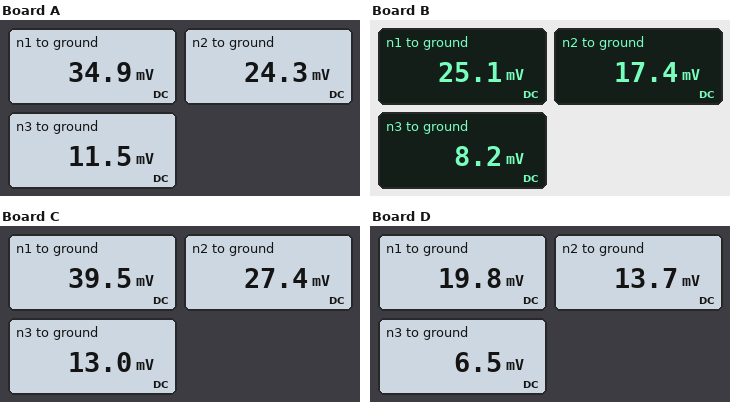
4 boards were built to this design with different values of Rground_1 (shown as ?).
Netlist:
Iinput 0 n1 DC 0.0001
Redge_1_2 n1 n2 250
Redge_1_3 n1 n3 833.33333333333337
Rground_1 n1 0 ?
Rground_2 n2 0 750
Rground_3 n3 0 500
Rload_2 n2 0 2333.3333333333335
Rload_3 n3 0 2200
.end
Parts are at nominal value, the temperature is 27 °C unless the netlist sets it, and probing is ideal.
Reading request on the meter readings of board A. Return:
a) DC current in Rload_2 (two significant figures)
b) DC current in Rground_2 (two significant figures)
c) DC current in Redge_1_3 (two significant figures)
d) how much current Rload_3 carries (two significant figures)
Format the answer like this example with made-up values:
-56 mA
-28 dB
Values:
10 µA
32 µA
28 µA
5.2 µA
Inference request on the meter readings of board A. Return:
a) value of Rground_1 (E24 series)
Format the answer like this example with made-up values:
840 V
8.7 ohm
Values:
1.2 kΩ
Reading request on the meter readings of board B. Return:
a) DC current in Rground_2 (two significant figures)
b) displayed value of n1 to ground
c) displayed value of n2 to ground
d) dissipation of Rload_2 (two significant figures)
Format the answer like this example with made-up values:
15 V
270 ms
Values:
23 µA
25.1 mV
17.4 mV
130 nW
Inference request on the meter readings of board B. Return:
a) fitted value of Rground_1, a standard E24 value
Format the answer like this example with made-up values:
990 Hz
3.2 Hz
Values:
510 Ω
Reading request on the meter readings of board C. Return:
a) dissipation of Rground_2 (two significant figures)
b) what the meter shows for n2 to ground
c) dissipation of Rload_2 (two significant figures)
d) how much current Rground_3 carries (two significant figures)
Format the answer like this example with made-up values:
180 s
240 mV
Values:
1.0 µW
27.4 mV
320 nW
26 µA
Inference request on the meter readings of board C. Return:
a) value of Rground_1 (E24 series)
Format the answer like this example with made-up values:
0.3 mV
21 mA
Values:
2 kΩ
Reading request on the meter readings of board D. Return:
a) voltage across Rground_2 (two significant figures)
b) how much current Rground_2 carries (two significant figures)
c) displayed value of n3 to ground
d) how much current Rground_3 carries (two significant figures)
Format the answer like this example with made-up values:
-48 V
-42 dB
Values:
14 mV
18 µA
6.5 mV
13 µA
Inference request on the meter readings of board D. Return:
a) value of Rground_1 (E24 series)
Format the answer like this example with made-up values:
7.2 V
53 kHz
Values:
330 Ω
